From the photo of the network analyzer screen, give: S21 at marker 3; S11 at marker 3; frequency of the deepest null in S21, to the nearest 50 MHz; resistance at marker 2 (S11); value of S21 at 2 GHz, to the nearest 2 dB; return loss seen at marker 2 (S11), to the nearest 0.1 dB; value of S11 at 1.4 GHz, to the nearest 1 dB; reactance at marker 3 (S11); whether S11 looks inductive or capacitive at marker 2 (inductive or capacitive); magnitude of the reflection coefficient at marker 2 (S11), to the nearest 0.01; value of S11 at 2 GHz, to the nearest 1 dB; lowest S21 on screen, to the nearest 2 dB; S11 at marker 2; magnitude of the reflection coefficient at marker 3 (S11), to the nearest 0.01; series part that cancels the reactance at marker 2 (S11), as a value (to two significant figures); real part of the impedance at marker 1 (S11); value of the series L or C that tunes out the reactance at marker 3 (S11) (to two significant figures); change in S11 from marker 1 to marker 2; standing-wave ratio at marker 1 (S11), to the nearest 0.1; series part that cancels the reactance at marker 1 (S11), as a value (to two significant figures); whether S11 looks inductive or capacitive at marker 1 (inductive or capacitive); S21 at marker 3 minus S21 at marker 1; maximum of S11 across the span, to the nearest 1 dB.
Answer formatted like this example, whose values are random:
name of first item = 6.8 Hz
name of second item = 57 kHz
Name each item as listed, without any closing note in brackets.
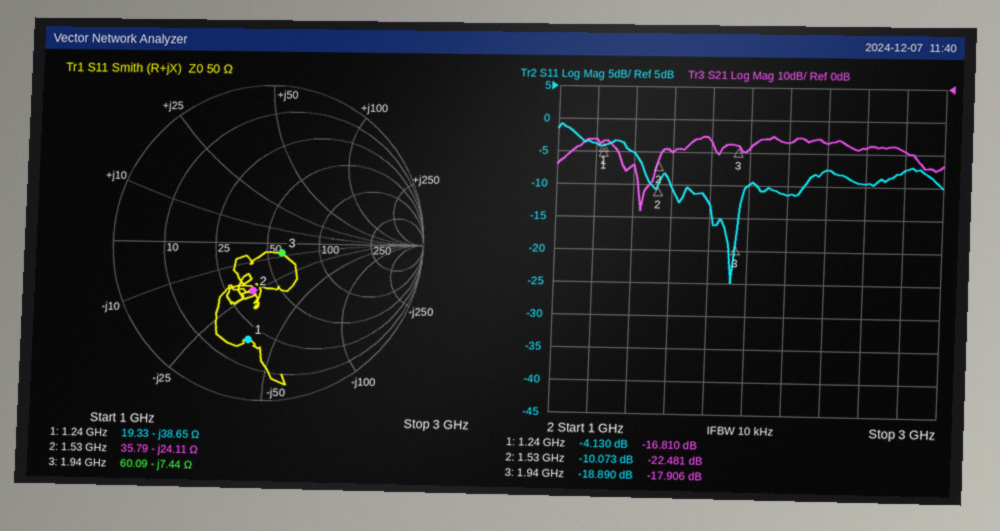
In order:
S21 at marker 3 = -17.906 dB
S11 at marker 3 = -18.890 dB
frequency of the deepest null in S21, to the nearest 50 MHz = 1.45 GHz
resistance at marker 2 = 35.79 Ω
value of S21 at 2 GHz, to the nearest 2 dB = -18 dB
return loss seen at marker 2 (S11), to the nearest 0.1 dB = 10.1 dB
value of S11 at 1.4 GHz, to the nearest 1 dB = -5 dB
reactance at marker 3 = -7.44 Ω
whether S11 looks inductive or capacitive at marker 2 = capacitive
magnitude of the reflection coefficient at marker 2 (S11), to the nearest 0.01 = 0.31
value of S11 at 2 GHz, to the nearest 1 dB = -10 dB
lowest S21 on screen, to the nearest 2 dB = -38 dB
S11 at marker 2 = -10.073 dB
magnitude of the reflection coefficient at marker 3 (S11), to the nearest 0.01 = 0.11
series part that cancels the reactance at marker 2 (S11), as a value = 2.5 nH
real part of the impedance at marker 1 = 19.33 Ω
value of the series L or C that tunes out the reactance at marker 3 (S11) = 610 pH
change in S11 from marker 1 to marker 2 = -5.943 dB
standing-wave ratio at marker 1 (S11), to the nearest 0.1 = 4.3
series part that cancels the reactance at marker 1 (S11), as a value = 5.0 nH
whether S11 looks inductive or capacitive at marker 1 = capacitive
S21 at marker 3 minus S21 at marker 1 = -1.096 dB
maximum of S11 across the span, to the nearest 1 dB = -1 dB
